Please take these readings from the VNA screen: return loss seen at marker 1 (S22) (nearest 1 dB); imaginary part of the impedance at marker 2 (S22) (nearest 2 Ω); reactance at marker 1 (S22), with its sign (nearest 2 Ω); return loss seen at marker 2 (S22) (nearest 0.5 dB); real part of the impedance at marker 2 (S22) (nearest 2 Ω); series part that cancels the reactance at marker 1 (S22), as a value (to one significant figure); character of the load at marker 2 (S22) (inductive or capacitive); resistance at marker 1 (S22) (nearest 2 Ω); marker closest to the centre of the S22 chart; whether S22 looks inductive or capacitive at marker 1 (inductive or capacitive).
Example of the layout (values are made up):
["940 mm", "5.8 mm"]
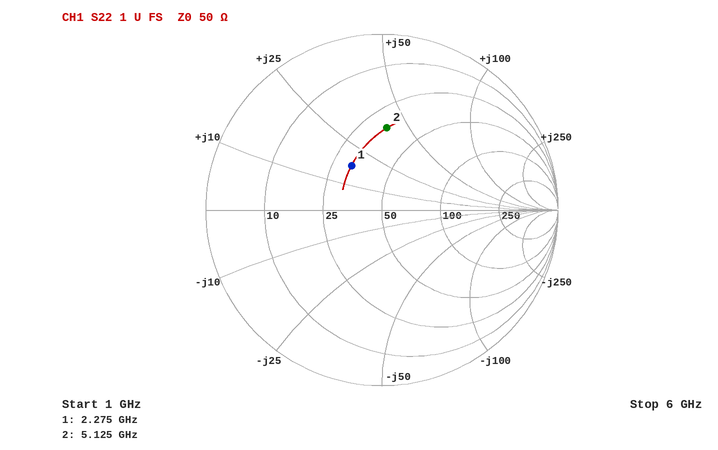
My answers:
["10 dB", "+40 Ω", "+18 Ω", "6.5 dB", "34 Ω", "4 pF", "inductive", "32 Ω", "marker 1", "inductive"]
